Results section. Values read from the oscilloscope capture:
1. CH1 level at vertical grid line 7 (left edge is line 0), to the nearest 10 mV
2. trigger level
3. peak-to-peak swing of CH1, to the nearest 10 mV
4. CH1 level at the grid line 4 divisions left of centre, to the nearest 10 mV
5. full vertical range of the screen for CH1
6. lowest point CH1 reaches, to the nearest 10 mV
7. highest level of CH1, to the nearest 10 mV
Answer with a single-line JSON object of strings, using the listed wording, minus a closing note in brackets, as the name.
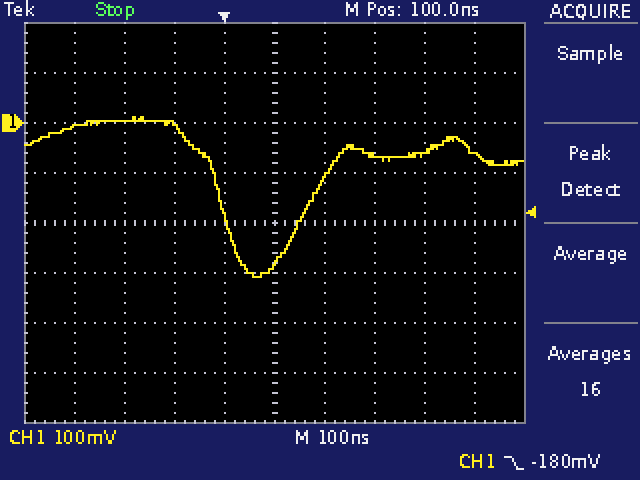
{"CH1 level at vertical grid line 7 (left edge is line 0), to the nearest 10 mV": "-60 mV", "trigger level": "-180 mV", "peak-to-peak swing of CH1, to the nearest 10 mV": "320 mV", "CH1 level at the grid line 4 divisions left of centre, to the nearest 10 mV": "-10 mV", "full vertical range of the screen for CH1": "800 mV", "lowest point CH1 reaches, to the nearest 10 mV": "-310 mV", "highest level of CH1, to the nearest 10 mV": "10 mV"}
